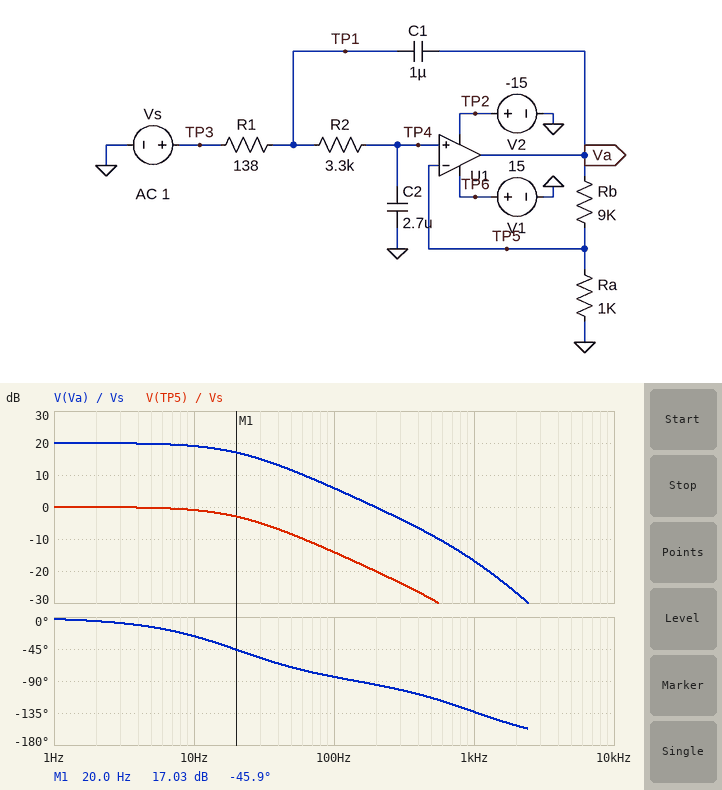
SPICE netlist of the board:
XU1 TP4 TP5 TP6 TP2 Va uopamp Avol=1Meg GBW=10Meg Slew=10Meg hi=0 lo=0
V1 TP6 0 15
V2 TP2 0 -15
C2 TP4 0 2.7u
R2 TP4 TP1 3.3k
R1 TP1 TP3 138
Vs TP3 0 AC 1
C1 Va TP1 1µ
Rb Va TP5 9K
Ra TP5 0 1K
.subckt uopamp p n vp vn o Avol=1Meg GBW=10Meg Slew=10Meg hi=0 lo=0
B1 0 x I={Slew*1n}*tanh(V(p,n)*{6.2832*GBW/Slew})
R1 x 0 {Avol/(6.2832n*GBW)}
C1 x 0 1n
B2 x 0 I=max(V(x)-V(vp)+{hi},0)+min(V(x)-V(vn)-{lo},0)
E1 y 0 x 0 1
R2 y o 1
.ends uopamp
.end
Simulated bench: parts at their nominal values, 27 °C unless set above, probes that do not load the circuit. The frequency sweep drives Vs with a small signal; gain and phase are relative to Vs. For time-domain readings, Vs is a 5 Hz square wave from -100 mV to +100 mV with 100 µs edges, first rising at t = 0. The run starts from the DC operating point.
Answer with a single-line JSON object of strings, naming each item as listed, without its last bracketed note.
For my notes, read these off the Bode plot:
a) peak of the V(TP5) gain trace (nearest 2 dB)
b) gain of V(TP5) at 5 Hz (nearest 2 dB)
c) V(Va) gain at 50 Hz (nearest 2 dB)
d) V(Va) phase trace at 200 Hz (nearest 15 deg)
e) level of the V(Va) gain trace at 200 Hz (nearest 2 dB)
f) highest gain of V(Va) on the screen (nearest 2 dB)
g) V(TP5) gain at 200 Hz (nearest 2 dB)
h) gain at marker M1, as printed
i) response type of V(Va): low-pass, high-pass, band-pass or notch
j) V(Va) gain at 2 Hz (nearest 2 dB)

{"peak of the V(TP5) gain trace": "0 dB", "gain of V(TP5) at 5 Hz": "0 dB", "V(Va) gain at 50 Hz": "12 dB", "V(Va) phase trace at 200 Hz": "-90 deg", "level of the V(Va) gain trace at 200 Hz": "0 dB", "highest gain of V(Va) on the screen": "20 dB", "V(TP5) gain at 200 Hz": "-20 dB", "gain at marker M1, as printed": "17.03 dB", "response type of V(Va): low-pass, high-pass, band-pass or notch": "low-pass", "V(Va) gain at 2 Hz": "20 dB"}
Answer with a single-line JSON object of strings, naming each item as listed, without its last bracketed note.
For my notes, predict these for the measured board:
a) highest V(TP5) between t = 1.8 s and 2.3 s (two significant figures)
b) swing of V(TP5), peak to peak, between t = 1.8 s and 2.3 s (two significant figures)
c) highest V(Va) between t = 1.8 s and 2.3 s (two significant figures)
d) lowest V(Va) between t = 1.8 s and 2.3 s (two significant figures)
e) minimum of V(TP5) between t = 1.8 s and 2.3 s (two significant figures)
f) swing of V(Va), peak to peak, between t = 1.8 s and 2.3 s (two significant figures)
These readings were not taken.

{"highest V(TP5) between t = 1.8 s and 2.3 s": "100 mV", "swing of V(TP5), peak to peak, between t = 1.8 s and 2.3 s": "200 mV", "highest V(Va) between t = 1.8 s and 2.3 s": "1.0 V", "lowest V(Va) between t = 1.8 s and 2.3 s": "-1.0 V", "minimum of V(TP5) between t = 1.8 s and 2.3 s": "-100 mV", "swing of V(Va), peak to peak, between t = 1.8 s and 2.3 s": "2.0 V"}
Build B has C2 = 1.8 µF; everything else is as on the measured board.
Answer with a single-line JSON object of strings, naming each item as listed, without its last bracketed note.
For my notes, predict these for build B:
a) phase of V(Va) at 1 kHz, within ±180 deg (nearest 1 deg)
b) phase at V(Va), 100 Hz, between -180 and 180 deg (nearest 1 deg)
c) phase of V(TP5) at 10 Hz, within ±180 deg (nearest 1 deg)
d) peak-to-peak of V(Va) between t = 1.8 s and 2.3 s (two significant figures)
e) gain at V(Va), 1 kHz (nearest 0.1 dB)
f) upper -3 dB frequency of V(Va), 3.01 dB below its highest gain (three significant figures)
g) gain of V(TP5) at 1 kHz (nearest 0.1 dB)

{"phase of V(Va) at 1 kHz, within ±180 deg": "-135 deg", "phase at V(Va), 100 Hz, between -180 and 180 deg": "-78 deg", "phase of V(TP5) at 10 Hz, within ±180 deg": "-17 deg", "peak-to-peak of V(Va) between t = 1.8 s and 2.3 s": "2.0 V", "gain at V(Va), 1 kHz": "-12.9 dB", "upper -3 dB frequency of V(Va), 3.01 dB below its highest gain": "33.3 Hz", "gain of V(TP5) at 1 kHz": "-32.9 dB"}
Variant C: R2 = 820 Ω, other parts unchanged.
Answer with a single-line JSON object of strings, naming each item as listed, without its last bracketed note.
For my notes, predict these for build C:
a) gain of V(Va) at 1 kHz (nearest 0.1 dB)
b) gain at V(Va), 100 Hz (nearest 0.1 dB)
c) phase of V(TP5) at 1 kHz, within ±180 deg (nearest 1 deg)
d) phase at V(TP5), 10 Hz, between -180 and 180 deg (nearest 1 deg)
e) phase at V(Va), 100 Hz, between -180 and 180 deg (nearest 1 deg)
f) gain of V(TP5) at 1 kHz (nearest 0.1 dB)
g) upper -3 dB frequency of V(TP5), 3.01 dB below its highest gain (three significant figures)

{"gain of V(Va) at 1 kHz": "-2.9 dB", "gain at V(Va), 100 Hz": "18.3 dB", "phase of V(TP5) at 1 kHz, within ±180 deg": "-143 deg", "phase at V(TP5), 10 Hz, between -180 and 180 deg": "-5 deg", "phase at V(Va), 100 Hz, between -180 and 180 deg": "-44 deg", "gain of V(TP5) at 1 kHz": "-22.9 dB", "upper -3 dB frequency of V(TP5), 3.01 dB below its highest gain": "141 Hz"}
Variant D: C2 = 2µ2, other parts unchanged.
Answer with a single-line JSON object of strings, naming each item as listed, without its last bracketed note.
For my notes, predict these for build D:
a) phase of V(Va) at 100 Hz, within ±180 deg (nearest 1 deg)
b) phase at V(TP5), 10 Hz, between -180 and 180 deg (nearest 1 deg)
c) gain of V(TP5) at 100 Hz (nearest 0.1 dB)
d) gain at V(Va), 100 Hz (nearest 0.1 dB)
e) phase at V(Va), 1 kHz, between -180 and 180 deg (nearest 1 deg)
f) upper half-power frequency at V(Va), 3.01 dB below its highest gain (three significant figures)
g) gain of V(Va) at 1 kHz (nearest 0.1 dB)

{"phase of V(Va) at 100 Hz, within ±180 deg": "-81 deg", "phase at V(TP5), 10 Hz, between -180 and 180 deg": "-22 deg", "gain of V(TP5) at 100 Hz": "-12.1 dB", "gain at V(Va), 100 Hz": "7.9 dB", "phase at V(Va), 1 kHz, between -180 and 180 deg": "-134 deg", "upper half-power frequency at V(Va), 3.01 dB below its highest gain": "25.8 Hz", "gain of V(Va) at 1 kHz": "-14.9 dB"}
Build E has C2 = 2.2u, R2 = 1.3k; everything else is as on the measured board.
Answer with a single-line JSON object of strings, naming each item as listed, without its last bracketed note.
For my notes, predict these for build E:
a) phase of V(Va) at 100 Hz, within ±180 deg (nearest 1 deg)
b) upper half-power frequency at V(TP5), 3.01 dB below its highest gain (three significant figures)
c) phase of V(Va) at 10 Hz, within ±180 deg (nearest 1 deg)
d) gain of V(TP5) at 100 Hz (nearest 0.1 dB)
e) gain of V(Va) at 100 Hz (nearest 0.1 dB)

{"phase of V(Va) at 100 Hz, within ±180 deg": "-55 deg", "upper half-power frequency at V(TP5), 3.01 dB below its highest gain": "92.6 Hz", "phase of V(Va) at 10 Hz, within ±180 deg": "-7 deg", "gain of V(TP5) at 100 Hz": "-3.4 dB", "gain of V(Va) at 100 Hz": "16.6 dB"}
